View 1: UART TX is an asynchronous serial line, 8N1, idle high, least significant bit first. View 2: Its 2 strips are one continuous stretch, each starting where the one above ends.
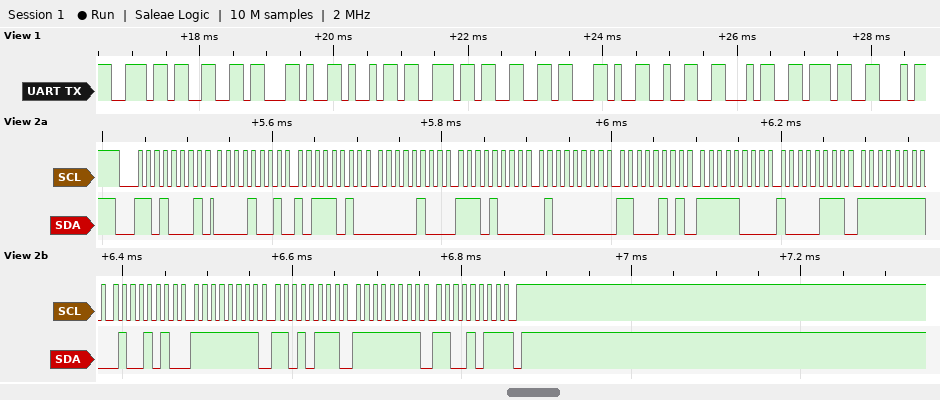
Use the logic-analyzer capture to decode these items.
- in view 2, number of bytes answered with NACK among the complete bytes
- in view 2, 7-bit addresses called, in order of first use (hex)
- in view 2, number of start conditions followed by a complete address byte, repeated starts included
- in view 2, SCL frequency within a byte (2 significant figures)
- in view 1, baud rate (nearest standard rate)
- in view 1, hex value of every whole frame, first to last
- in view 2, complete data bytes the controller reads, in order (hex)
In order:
1
0x68
1
100 kHz
9600 baud
6E 66 2C 69 6E 66 2C 32 34 37
09 BA 04 E8 40 C5 F8 87 FF 4A FF D7 FF CB
